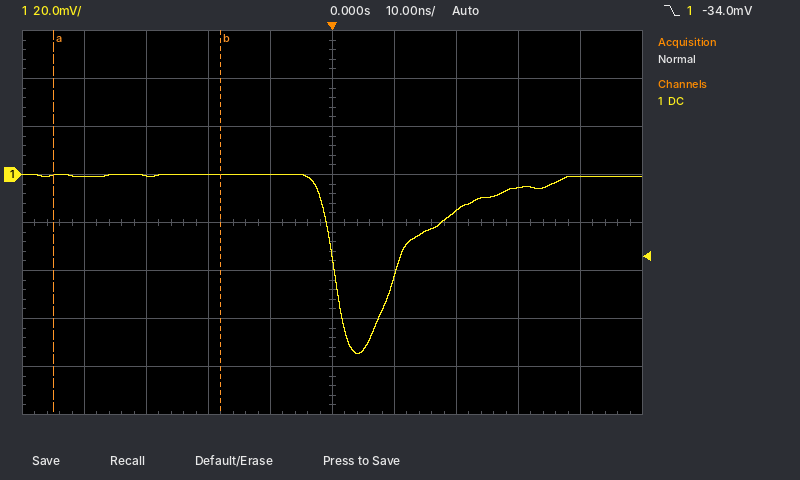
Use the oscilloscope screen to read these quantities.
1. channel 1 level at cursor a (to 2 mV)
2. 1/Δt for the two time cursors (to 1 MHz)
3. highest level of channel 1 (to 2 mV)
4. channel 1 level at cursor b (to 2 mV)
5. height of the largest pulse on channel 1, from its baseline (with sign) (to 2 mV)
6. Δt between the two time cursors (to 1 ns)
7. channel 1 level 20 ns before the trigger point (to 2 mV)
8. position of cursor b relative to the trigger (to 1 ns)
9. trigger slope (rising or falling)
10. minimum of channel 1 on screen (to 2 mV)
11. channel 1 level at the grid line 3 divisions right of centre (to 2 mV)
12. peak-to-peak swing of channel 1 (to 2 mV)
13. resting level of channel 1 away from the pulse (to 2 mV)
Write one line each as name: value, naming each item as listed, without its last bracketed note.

channel 1 level at cursor a: 0 mV
1/Δt for the two time cursors: 37 MHz
highest level of channel 1: 0 mV
channel 1 level at cursor b: 0 mV
height of the largest pulse on channel 1, from its baseline (with sign): -74 mV
Δt between the two time cursors: 27 ns
channel 1 level 20 ns before the trigger point: 0 mV
position of cursor b relative to the trigger: -18 ns
trigger slope: falling
minimum of channel 1 on screen: -74 mV
channel 1 level at the grid line 3 divisions right of centre: -6 mV
peak-to-peak swing of channel 1: 74 mV
resting level of channel 1 away from the pulse: 0 mV
